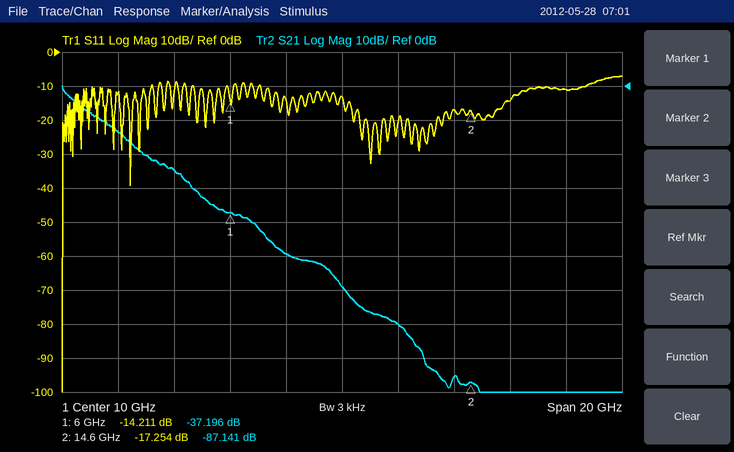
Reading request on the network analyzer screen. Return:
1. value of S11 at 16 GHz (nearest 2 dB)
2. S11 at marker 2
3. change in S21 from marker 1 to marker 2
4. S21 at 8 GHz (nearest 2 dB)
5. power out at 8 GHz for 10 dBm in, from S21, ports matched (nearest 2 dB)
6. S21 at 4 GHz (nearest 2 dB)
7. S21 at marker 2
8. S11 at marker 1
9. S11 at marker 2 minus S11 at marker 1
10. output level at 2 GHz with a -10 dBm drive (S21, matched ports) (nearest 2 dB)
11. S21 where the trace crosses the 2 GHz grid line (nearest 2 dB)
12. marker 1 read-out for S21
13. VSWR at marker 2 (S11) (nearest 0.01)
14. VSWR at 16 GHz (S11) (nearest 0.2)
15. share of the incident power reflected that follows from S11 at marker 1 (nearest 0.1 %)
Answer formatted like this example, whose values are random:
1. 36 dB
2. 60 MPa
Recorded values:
1. -14 dB
2. -17.254 dB
3. -49.945 dB
4. -50 dB
5. -40 dBm
6. -24 dB
7. -87.141 dB
8. -14.211 dB
9. -3.043 dB
10. -24 dBm
11. -14 dB
12. -37.196 dB
13. 1.32
14. 1.4
15. 3.8 %
